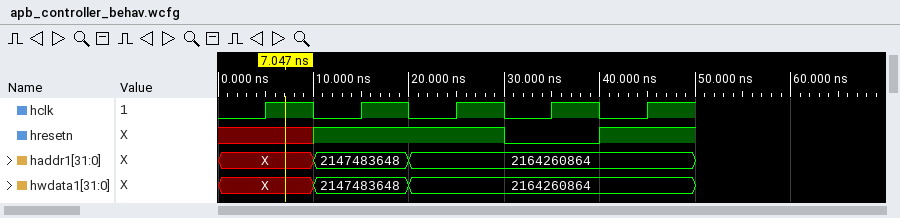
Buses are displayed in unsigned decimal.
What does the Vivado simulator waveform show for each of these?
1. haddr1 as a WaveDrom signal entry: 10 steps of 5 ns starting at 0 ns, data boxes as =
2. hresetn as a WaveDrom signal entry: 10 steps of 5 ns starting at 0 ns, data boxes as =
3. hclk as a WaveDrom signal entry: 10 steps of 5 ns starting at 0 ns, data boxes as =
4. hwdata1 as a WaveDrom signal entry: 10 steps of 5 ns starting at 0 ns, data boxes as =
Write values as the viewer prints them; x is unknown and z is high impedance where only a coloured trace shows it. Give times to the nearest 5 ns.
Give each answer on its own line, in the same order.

{name: 'haddr1', wave: 'x.=.=.....', data: '2147483648 2164260864'}
{name: 'hresetn', wave: 'x.1...0.1.'}
{name: 'hclk', wave: '0101010101'}
{name: 'hwdata1', wave: 'x.=.=.....', data: '2147483648 2164260864'}
